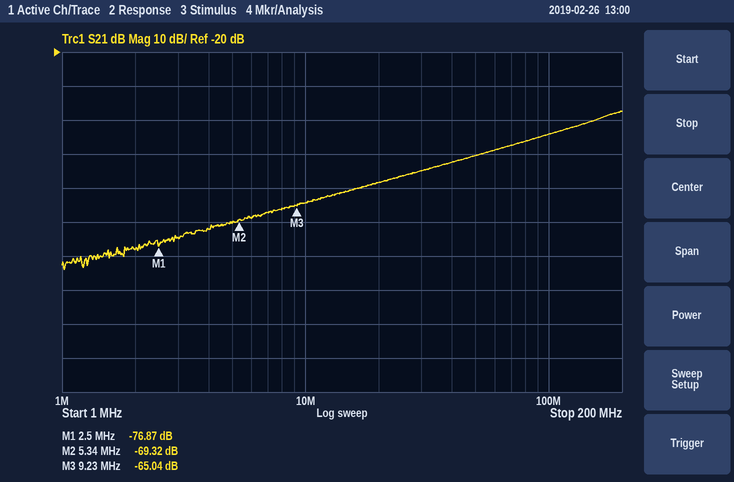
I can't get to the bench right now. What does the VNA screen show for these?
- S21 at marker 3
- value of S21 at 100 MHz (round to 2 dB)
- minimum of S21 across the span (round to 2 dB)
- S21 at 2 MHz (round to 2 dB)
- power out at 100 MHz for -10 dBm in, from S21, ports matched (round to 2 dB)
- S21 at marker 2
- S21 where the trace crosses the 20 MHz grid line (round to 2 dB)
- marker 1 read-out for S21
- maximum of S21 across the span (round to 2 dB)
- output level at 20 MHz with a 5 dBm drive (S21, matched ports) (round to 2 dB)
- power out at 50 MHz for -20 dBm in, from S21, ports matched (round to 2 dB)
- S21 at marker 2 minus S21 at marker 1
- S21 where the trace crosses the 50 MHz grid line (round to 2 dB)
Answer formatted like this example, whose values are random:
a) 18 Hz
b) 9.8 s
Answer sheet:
a) -65.04 dB
b) -44 dB
c) -84 dB
d) -78 dB
e) -54 dBm
f) -69.32 dB
g) -58 dB
h) -76.87 dB
i) -38 dB
j) -54 dBm
k) -70 dBm
l) 7.55 dB
m) -50 dB
